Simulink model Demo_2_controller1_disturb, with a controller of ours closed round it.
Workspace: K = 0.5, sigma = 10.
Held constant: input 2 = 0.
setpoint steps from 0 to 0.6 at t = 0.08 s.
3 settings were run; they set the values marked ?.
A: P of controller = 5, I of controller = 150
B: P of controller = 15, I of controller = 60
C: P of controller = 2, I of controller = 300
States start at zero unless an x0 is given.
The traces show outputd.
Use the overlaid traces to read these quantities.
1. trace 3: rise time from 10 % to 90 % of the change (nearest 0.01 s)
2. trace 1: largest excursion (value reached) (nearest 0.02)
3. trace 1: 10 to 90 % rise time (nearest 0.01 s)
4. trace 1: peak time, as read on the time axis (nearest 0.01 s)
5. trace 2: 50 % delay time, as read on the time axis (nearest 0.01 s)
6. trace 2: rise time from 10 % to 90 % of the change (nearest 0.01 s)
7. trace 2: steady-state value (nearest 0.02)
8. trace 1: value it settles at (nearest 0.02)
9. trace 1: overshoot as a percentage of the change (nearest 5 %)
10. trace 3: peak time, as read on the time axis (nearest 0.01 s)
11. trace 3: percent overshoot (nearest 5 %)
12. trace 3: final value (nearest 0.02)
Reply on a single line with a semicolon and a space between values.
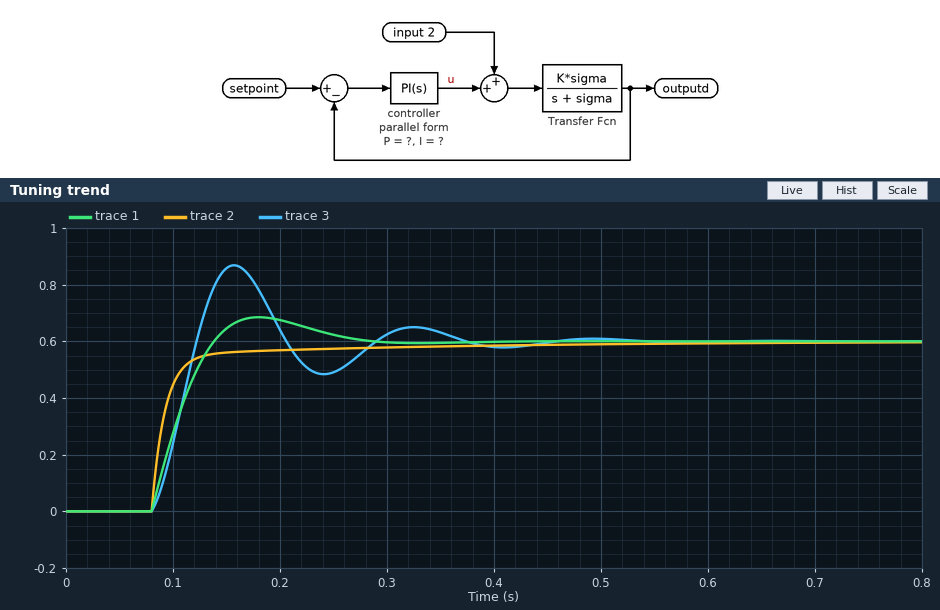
0.03 s; 0.68; 0.04 s; 0.18 s; 0.09 s; 0.04 s; 0.60; 0.60; 15 %; 0.16 s; 45 %; 0.60
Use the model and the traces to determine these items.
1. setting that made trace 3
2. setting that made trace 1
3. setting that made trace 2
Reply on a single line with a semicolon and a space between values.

C; A; B
